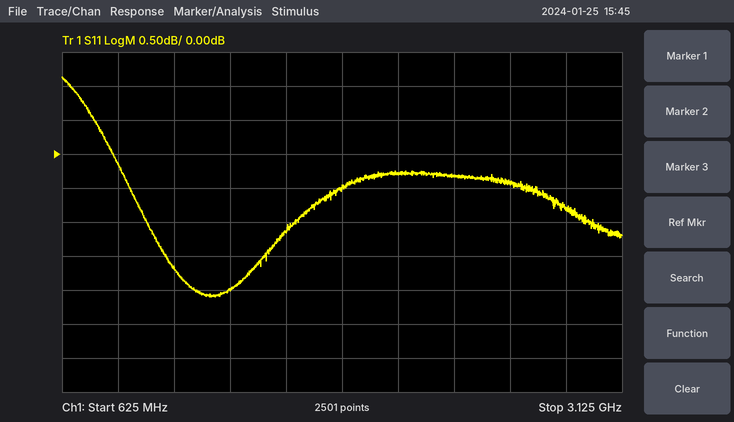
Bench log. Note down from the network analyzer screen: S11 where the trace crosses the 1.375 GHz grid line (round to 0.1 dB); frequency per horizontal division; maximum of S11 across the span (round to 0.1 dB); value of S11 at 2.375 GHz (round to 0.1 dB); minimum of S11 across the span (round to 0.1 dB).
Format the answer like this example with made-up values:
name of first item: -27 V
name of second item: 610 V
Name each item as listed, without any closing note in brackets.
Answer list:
S11 where the trace crosses the 1.375 GHz grid line: -2.0 dB
frequency per horizontal division: 250 MHz
maximum of S11 across the span: 1.1 dB
value of S11 at 2.375 GHz: -0.3 dB
minimum of S11 across the span: -2.1 dB
